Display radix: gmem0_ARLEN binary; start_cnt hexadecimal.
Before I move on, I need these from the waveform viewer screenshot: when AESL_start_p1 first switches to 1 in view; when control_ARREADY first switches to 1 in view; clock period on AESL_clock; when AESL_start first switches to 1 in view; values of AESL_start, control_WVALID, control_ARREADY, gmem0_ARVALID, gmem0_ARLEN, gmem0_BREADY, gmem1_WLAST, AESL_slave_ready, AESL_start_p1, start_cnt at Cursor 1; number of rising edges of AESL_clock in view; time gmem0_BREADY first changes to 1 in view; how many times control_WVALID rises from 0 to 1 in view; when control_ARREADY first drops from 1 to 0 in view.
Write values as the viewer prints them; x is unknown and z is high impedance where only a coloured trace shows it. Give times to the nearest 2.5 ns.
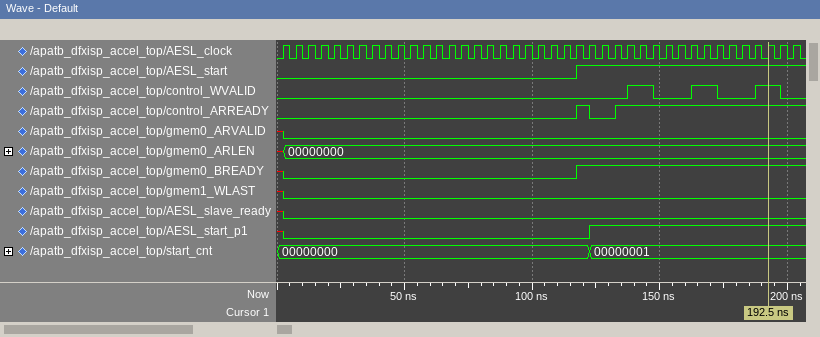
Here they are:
122.5 ns
117.5 ns
5 ns
117.5 ns
AESL_start=1, control_WVALID=1, control_ARREADY=1, gmem0_ARVALID=0, gmem0_ARLEN=00000000, gmem0_BREADY=1, gmem1_WLAST=0, AESL_slave_ready=0, AESL_start_p1=1, start_cnt=00000001
41
117.5 ns
3
122.5 ns
